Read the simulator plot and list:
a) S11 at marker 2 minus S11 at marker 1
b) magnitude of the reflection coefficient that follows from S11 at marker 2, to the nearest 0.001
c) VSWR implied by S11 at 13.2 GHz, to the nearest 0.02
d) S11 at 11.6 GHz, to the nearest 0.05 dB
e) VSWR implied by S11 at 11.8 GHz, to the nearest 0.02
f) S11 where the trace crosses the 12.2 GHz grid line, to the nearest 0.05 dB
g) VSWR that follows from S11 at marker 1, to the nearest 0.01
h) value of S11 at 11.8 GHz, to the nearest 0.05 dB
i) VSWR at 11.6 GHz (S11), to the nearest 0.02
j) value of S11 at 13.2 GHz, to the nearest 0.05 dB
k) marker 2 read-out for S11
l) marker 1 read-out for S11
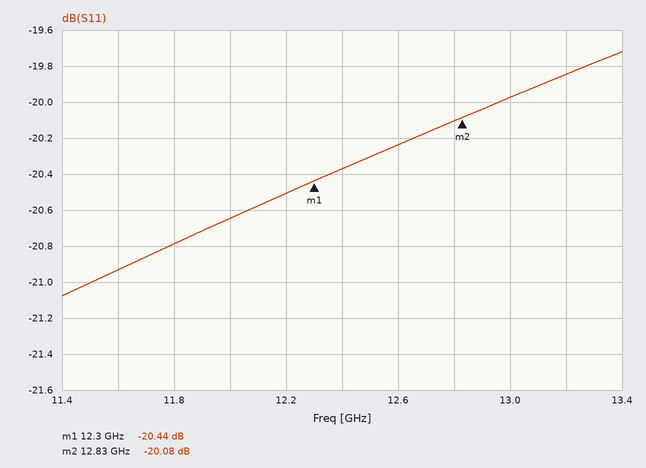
0.36 dB
0.099
1.22
-20.95 dB
1.20
-20.50 dB
1.21
-20.80 dB
1.20
-19.85 dB
-20.08 dB
-20.44 dB
